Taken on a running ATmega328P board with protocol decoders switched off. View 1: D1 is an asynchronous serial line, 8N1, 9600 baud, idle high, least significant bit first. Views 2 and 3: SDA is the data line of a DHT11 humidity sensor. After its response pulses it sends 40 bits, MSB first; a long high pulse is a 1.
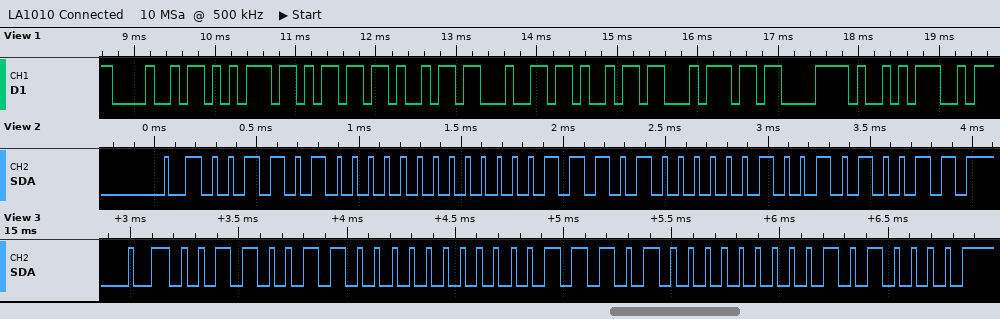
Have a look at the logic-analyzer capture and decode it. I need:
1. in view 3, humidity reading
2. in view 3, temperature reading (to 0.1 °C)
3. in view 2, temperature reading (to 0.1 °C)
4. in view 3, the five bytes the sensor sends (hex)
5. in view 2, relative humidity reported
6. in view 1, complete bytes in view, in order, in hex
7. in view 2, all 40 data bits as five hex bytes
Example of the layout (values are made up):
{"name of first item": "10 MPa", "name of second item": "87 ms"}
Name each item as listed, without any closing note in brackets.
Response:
{"in view 3, humidity reading": "51 %", "in view 3, temperature reading": "29.0 °C", "in view 2, temperature reading": "29.2 °C", "in view 3, the five bytes the sensor sends": "33 00 1D 00 50", "in view 2, relative humidity reported": "52 %", "in view 1, complete bytes in view, in order, in hex": "48 75 6D 69 64 69 74 C3 A9", "in view 2, all 40 data bits as five hex bytes": "34 00 1D 02 53"}
